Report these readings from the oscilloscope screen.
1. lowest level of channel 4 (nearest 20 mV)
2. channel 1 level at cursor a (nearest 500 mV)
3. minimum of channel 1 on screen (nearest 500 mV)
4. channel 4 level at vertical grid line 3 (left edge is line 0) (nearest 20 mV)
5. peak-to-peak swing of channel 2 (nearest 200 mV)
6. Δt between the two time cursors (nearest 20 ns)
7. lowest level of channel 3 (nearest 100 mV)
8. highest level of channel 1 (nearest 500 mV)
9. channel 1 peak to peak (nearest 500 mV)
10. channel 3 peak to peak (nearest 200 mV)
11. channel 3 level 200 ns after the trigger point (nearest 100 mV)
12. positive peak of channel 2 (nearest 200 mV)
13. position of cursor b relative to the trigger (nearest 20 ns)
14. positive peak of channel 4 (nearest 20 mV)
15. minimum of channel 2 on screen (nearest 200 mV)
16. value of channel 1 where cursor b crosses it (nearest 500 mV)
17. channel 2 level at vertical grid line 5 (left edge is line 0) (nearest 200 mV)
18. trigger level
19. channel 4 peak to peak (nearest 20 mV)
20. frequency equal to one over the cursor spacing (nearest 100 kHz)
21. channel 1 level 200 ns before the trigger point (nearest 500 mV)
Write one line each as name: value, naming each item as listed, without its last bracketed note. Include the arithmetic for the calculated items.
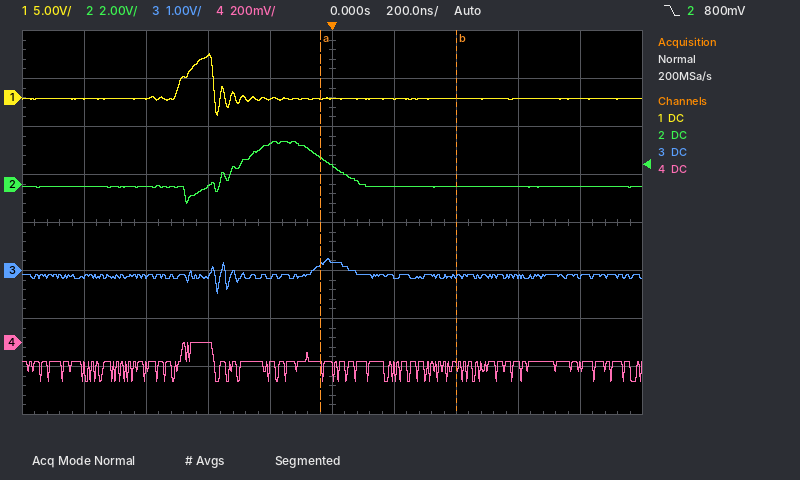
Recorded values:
lowest level of channel 4: -160 mV
channel 1 level at cursor a: 0.0 V
minimum of channel 1 on screen: -2.0 V
channel 4 level at vertical grid line 3 (left edge is line 0): 0 mV
peak-to-peak swing of channel 2: 1.8 V − (-800 mV) = 2.6 V
Δt between the two time cursors: 440 ns
lowest level of channel 3: -500 mV
highest level of channel 1: 4.5 V
channel 1 peak to peak: 4.5 V − (-2.0 V) = 6.5 V
channel 3 peak to peak: 800 mV
channel 3 level 200 ns after the trigger point: -100 mV
positive peak of channel 2: 1.8 V
position of cursor b relative to the trigger: +400 ns
positive peak of channel 4: 0 mV
minimum of channel 2 on screen: -800 mV
value of channel 1 where cursor b crosses it: 0.0 V
channel 2 level at vertical grid line 5 (left edge is line 0): 800 mV
trigger level: 800 mV
channel 4 peak to peak: 0 mV − (-160 mV) = 160 mV
frequency equal to one over the cursor spacing: 1 / 440 ns ≈ 2.3 MHz
channel 1 level 200 ns before the trigger point: 0.0 V
